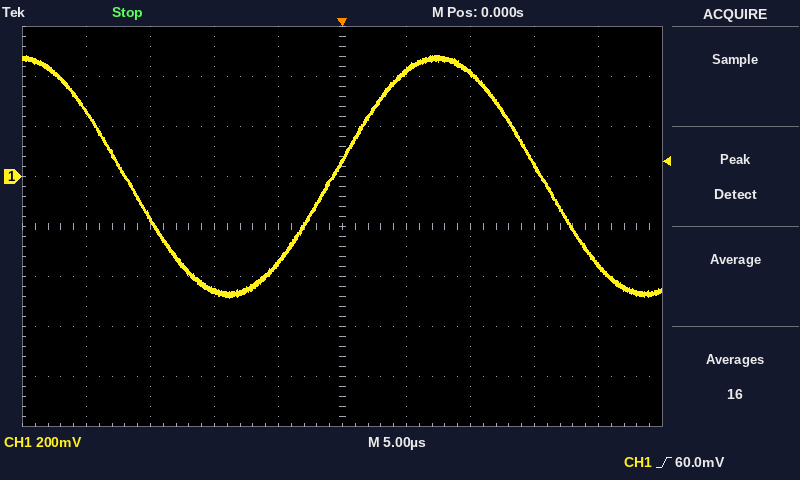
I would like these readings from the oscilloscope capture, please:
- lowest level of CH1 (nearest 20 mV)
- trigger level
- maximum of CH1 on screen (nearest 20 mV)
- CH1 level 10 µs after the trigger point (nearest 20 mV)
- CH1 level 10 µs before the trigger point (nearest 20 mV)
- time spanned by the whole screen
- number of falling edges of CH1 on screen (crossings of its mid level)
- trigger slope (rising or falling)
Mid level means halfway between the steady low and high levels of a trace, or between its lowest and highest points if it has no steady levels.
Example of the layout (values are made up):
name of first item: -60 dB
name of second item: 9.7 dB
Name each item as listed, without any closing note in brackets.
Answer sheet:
lowest level of CH1: -480 mV
trigger level: 60.0 mV
maximum of CH1 on screen: 480 mV
CH1 level 10 µs after the trigger point: 420 mV
CH1 level 10 µs before the trigger point: -460 mV
time spanned by the whole screen: 50 µs
number of falling edges of CH1 on screen: 2
trigger slope: rising
